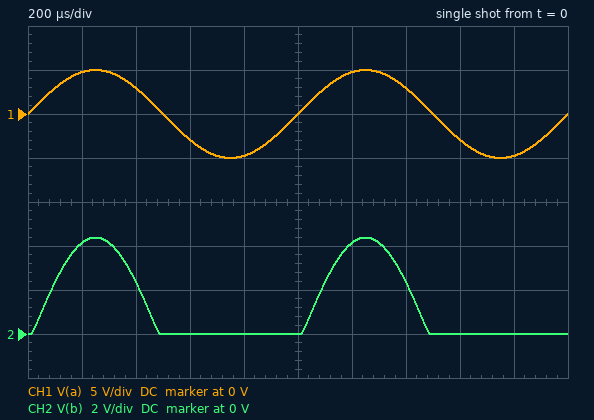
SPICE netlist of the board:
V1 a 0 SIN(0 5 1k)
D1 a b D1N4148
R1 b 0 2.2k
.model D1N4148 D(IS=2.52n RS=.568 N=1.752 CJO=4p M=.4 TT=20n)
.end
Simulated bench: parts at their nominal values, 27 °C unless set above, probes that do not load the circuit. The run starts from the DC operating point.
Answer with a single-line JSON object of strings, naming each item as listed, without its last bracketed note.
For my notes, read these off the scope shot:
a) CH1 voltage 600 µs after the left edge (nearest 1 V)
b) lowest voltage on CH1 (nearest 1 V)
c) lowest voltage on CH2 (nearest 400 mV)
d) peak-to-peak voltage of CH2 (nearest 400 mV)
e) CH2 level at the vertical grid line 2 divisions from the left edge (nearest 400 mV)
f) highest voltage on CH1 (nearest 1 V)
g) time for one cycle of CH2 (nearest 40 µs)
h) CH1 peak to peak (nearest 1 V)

{"CH1 voltage 600 µs after the left edge": "-3 V", "lowest voltage on CH1": "-5 V", "lowest voltage on CH2": "0 V", "peak-to-peak voltage of CH2": "4.4 V", "CH2 level at the vertical grid line 2 divisions from the left edge": "2.4 V", "highest voltage on CH1": "5 V", "time for one cycle of CH2": "1.00 ms", "CH1 peak to peak": "10 V"}
